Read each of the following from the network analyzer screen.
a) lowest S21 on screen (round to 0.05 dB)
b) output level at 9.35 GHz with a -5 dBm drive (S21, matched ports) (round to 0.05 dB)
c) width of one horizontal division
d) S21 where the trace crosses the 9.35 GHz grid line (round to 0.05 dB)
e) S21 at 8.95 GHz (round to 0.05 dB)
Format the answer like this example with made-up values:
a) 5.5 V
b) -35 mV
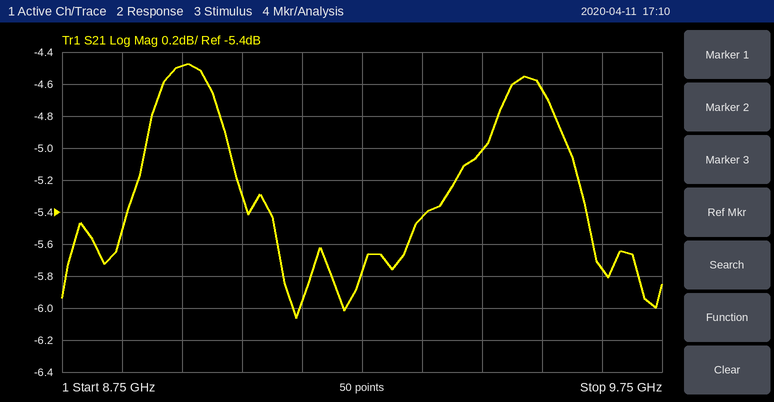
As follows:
a) -6.05 dB
b) -10.45 dBm
c) 100 MHz
d) -5.45 dB
e) -4.50 dB
